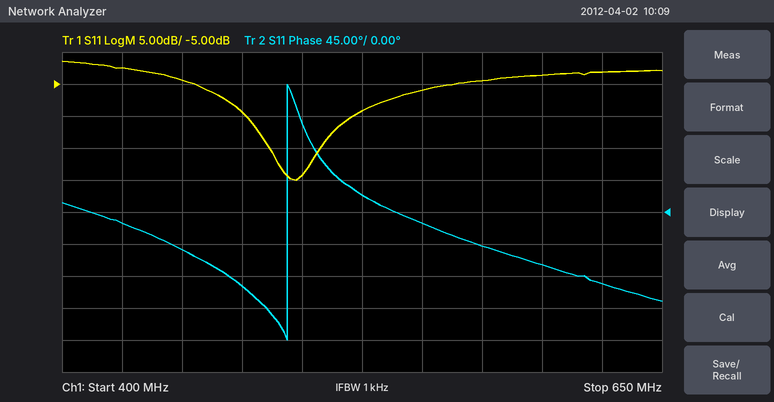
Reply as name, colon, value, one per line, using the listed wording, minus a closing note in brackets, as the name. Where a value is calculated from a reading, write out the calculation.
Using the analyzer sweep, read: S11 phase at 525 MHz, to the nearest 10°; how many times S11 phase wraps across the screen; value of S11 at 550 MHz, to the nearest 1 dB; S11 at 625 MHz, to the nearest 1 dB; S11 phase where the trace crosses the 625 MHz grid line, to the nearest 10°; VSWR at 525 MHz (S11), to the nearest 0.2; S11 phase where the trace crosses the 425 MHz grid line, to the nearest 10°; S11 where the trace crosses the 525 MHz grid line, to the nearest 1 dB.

S11 phase at 525 MHz, to the nearest 10°: 20°
how many times S11 phase wraps across the screen: 1
value of S11 at 550 MHz, to the nearest 1 dB: -6 dB
S11 at 625 MHz, to the nearest 1 dB: -3 dB
S11 phase where the trace crosses the 625 MHz grid line, to the nearest 10°: -100°
VSWR at 525 MHz (S11), to the nearest 0.2: |Γ| = 10^(-9/20) = 0.3548; VSWR = (1 + 0.3548)/(1 − 0.3548) ≈ 2.10, so 2.0 to the nearest 0.2
S11 phase where the trace crosses the 425 MHz grid line, to the nearest 10°: -20°
S11 where the trace crosses the 525 MHz grid line, to the nearest 1 dB: -9 dB
